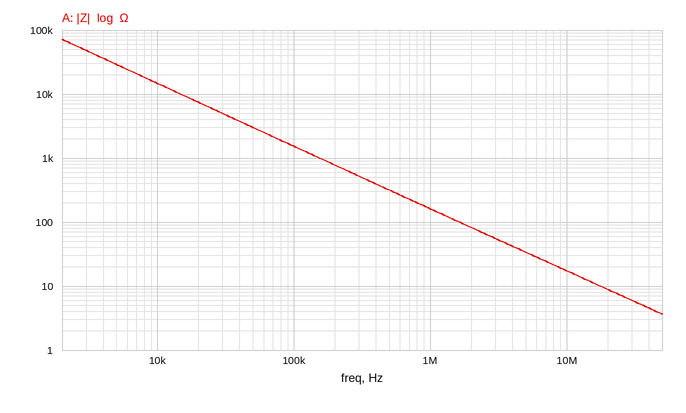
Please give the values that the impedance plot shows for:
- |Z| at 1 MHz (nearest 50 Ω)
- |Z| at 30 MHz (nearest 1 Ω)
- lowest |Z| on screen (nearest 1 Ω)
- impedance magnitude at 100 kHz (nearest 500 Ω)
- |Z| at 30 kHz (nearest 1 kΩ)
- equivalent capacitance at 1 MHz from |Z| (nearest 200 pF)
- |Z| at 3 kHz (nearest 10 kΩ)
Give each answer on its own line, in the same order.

150 Ω
6 Ω
4 Ω
1.5 kΩ
5 kΩ
1.0 nF
50 kΩ
